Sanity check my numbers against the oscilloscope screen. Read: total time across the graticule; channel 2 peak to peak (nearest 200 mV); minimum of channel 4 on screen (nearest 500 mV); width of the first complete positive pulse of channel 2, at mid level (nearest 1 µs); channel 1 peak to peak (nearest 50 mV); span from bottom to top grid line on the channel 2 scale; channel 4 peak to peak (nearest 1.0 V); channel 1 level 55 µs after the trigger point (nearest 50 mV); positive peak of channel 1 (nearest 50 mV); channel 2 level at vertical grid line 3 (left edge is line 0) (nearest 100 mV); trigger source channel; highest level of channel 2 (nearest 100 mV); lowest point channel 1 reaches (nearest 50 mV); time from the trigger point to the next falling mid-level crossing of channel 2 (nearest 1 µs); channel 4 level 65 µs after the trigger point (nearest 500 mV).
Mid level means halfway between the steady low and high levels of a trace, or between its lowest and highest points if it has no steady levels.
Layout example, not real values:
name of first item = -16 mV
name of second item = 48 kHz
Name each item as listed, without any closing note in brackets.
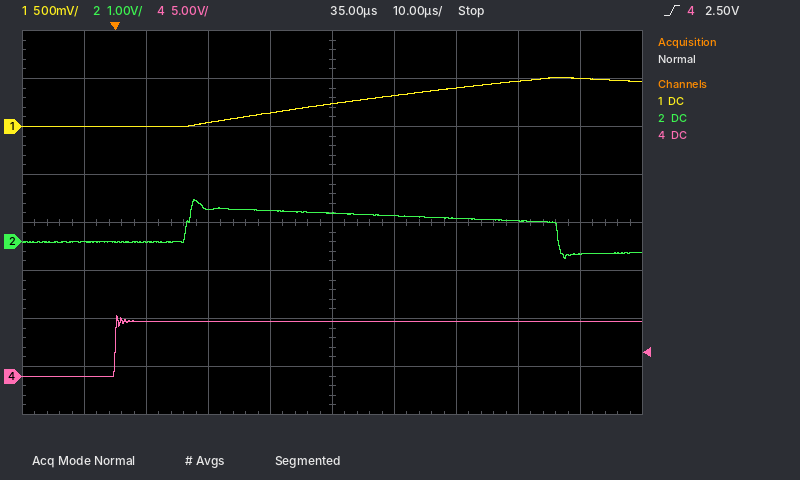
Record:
total time across the graticule = 100 µs
channel 2 peak to peak = 1.2 V
minimum of channel 4 on screen = 0.0 V
width of the first complete positive pulse of channel 2, at mid level = 60 µs
channel 1 peak to peak = 500 mV
span from bottom to top grid line on the channel 2 scale = 8 V
channel 4 peak to peak = 6.0 V
channel 1 level 55 µs after the trigger point = 400 mV
positive peak of channel 1 = 500 mV
channel 2 level at vertical grid line 3 (left edge is line 0) = 700 mV
trigger source channel = channel 4
highest level of channel 2 = 900 mV
lowest point channel 1 reaches = 0 mV
time from the trigger point to the next falling mid-level crossing of channel 2 = 71 µs
channel 4 level 65 µs after the trigger point = 5.5 V
